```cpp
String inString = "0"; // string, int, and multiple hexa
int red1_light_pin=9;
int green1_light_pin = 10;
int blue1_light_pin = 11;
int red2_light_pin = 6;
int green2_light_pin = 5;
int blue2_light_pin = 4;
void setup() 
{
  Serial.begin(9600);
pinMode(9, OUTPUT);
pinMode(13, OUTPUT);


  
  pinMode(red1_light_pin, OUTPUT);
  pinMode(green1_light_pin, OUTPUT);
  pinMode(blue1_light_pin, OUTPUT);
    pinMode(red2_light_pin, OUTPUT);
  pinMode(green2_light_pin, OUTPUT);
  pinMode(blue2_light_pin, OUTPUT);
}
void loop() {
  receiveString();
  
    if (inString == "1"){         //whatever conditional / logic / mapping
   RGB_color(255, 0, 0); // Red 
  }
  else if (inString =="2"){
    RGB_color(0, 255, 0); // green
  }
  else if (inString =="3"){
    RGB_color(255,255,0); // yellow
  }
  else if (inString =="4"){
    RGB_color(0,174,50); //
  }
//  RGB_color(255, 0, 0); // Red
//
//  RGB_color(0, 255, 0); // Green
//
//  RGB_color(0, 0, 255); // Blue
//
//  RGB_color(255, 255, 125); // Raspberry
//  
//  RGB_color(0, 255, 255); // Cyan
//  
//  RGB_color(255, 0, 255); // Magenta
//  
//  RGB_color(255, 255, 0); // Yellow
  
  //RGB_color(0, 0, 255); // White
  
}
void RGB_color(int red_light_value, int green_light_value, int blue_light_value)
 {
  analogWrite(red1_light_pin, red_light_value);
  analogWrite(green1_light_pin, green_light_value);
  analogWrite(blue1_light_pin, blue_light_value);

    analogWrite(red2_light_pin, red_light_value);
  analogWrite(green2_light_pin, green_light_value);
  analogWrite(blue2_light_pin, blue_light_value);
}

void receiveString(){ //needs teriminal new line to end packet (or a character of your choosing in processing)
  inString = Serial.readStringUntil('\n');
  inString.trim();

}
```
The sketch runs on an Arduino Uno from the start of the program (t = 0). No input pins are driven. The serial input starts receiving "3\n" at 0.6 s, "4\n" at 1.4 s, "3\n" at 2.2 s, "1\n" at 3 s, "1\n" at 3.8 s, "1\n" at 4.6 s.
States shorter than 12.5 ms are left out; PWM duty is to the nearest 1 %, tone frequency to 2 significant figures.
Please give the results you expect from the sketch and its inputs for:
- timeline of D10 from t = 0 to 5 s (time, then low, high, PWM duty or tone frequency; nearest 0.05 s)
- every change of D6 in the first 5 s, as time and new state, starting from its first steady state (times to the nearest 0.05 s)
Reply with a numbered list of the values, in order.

1. 0 s low; 0.6 s high; 1.4 s PWM 68 %; 2.2 s high; 3 s low
2. 0 s low; 0.6 s high; 1.4 s low; 2.2 s high
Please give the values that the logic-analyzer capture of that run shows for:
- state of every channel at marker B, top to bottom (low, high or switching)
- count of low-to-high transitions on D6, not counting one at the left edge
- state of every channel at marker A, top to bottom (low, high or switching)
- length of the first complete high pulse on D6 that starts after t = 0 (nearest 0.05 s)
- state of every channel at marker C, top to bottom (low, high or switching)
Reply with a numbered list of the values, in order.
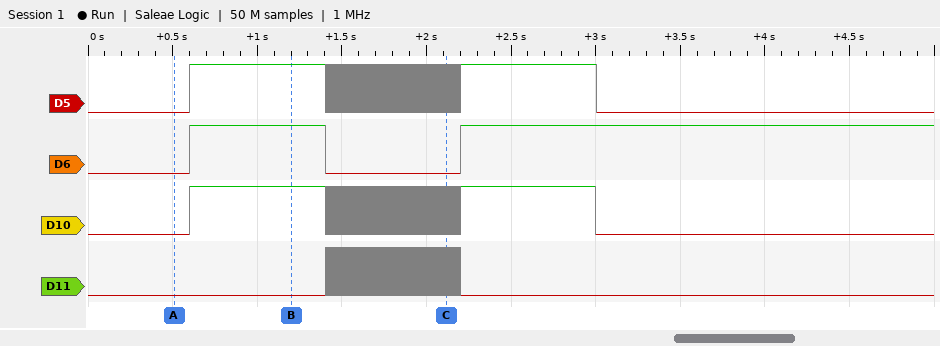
1. D5 high, D6 high, D10 high, D11 low
2. 2
3. D5 low, D6 low, D10 low, D11 low
4. 0.80 s
5. D5 switching, D6 low, D10 switching, D11 switching
